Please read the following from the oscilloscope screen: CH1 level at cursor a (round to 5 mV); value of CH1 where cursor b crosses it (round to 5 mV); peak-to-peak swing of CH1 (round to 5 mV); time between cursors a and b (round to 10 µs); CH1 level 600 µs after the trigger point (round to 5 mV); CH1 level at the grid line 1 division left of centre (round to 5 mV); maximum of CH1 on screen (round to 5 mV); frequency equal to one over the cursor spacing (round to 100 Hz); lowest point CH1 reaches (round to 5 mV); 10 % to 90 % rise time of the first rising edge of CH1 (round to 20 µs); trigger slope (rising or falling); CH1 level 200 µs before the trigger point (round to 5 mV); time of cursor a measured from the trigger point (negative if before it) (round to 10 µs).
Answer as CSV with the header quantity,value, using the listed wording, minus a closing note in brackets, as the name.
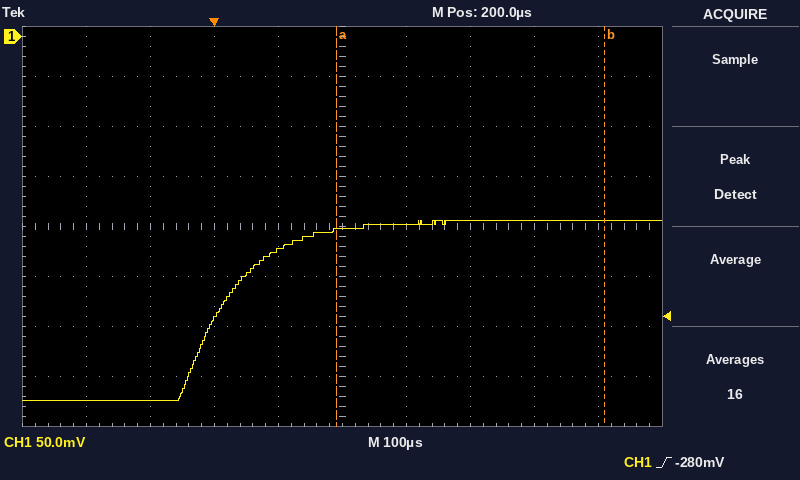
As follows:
quantity,value
CH1 level at cursor a,-195 mV
value of CH1 where cursor b crosses it,-185 mV
peak-to-peak swing of CH1,180 mV
time between cursors a and b,420 µs
CH1 level 600 µs after the trigger point,-185 mV
CH1 level at the grid line 1 division left of centre,-215 mV
maximum of CH1 on screen,-185 mV
frequency equal to one over the cursor spacing,2.4 kHz
lowest point CH1 reaches,-365 mV
10 % to 90 % rise time of the first rising edge of CH1,180 µs
trigger slope,rising
CH1 level 200 µs before the trigger point,-365 mV
time of cursor a measured from the trigger point (negative if before it),+190 µs
